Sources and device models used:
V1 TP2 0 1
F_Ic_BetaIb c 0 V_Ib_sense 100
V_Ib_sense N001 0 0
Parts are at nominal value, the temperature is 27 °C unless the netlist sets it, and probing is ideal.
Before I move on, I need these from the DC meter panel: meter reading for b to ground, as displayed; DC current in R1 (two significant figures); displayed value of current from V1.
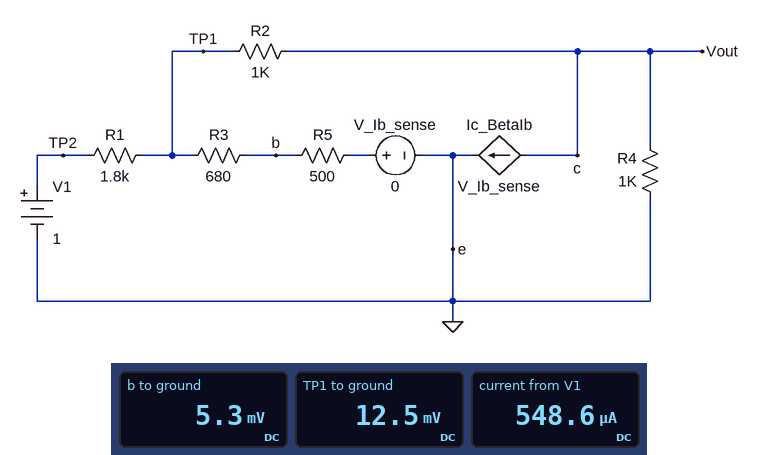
5.3 mV
550 µA
548.6 µA
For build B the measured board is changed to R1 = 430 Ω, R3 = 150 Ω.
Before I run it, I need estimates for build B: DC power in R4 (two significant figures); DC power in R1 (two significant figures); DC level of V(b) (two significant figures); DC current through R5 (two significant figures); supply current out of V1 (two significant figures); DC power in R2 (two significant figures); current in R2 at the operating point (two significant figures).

4.8 mW
2.2 mW
22 mV
44 µA
2.3 mA
4.9 mW
2.2 mA
